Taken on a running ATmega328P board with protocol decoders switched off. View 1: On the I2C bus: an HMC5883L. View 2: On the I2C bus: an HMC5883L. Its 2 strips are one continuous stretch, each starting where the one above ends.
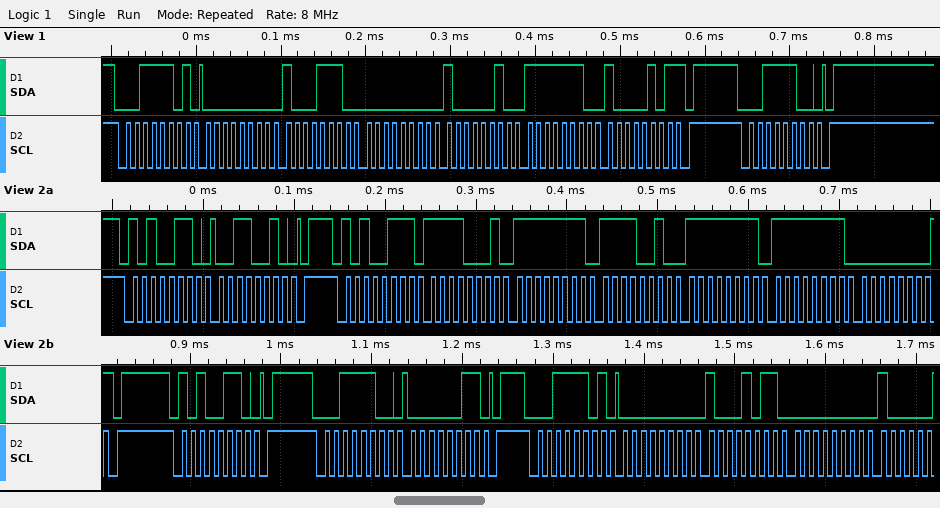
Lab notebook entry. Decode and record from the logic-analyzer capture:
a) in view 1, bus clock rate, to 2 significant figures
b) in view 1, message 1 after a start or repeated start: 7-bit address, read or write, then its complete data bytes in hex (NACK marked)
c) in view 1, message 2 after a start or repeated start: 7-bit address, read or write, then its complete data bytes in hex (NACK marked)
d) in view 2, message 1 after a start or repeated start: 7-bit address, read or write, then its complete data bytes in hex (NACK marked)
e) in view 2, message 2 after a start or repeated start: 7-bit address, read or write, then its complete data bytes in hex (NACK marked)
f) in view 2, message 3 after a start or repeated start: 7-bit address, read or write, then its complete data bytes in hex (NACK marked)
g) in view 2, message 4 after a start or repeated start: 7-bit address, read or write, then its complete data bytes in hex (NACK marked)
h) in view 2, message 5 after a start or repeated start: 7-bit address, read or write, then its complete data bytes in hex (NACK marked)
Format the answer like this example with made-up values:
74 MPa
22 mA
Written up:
100 kHz
0x1E read: 00 8E 00 82 FE 85 NACK
0x1E write
0x53 write: 32
0x53 read: F1 FF F2 FF FF 00 NACK
0x53 write
0x1E write: 03
0x1E read: 00 8B 00
